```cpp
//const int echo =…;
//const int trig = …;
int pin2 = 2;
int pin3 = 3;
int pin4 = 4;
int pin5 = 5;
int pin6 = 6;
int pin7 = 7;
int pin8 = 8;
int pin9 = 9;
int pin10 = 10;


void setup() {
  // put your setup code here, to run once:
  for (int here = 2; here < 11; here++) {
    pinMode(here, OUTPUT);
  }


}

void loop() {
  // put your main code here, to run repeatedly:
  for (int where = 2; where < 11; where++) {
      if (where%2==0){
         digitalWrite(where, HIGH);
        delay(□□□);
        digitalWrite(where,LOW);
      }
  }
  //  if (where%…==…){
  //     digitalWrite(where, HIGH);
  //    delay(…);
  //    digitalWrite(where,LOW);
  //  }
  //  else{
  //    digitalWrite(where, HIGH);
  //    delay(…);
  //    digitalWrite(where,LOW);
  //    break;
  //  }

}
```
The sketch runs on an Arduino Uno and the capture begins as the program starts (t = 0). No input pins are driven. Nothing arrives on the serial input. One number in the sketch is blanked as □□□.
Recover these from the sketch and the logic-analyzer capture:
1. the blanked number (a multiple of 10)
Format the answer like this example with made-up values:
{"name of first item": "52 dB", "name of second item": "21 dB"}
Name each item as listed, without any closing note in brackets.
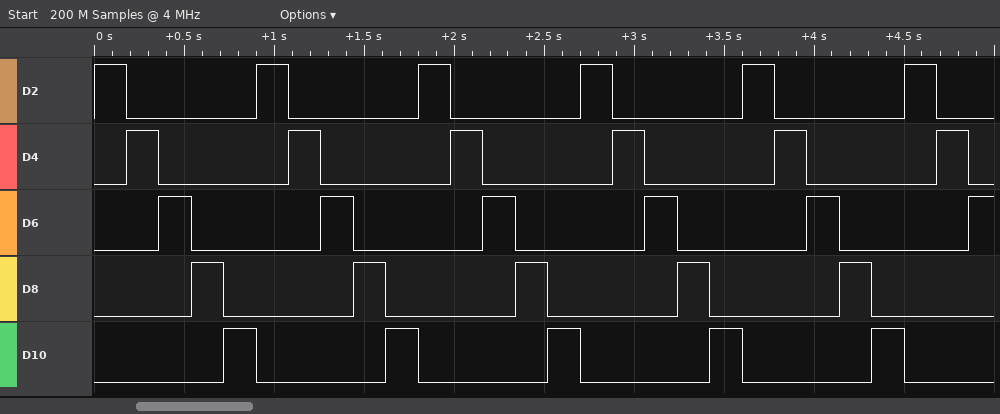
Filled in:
{"the blanked number": "180"}
